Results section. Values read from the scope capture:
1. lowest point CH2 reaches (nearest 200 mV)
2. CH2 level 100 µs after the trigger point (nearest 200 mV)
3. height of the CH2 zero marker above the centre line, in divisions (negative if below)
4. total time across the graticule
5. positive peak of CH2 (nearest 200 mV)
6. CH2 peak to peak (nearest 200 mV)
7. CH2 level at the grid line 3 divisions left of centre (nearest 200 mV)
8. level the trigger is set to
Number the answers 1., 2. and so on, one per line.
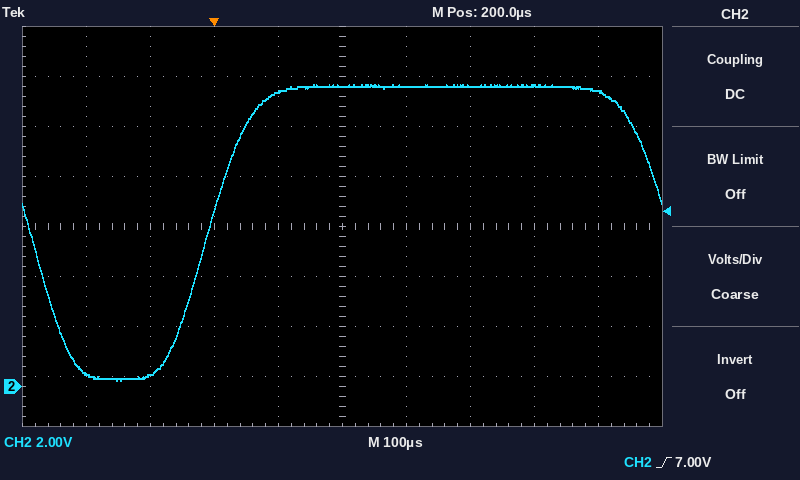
1. 200 mV
2. 11.8 V
3. -3.2 div
4. 1 ms
5. 12.0 V
6. 11.8 V
7. 400 mV
8. 7.00 V
